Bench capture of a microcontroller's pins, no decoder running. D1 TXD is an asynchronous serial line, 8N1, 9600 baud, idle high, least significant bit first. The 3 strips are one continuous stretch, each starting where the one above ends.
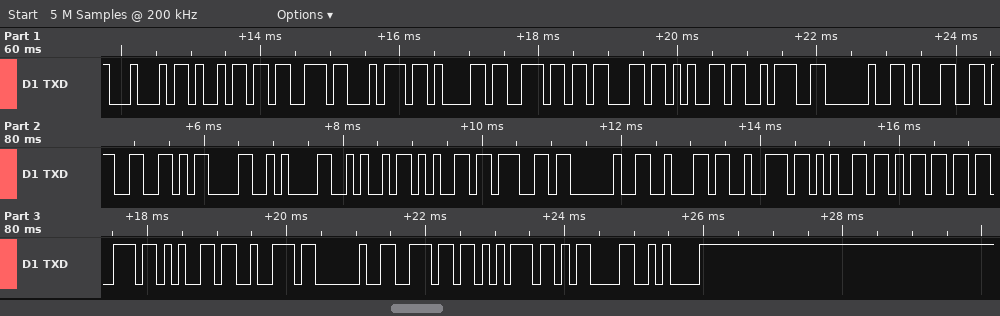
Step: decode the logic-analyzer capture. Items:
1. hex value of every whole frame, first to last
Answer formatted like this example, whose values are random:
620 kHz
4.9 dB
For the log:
44 69 73 74 61 6E 63 65 3A 20 31 33 0D 0A 4A 65 67 20 62 72 65 6D 73 65 72 20 6E 75 0D 0A
